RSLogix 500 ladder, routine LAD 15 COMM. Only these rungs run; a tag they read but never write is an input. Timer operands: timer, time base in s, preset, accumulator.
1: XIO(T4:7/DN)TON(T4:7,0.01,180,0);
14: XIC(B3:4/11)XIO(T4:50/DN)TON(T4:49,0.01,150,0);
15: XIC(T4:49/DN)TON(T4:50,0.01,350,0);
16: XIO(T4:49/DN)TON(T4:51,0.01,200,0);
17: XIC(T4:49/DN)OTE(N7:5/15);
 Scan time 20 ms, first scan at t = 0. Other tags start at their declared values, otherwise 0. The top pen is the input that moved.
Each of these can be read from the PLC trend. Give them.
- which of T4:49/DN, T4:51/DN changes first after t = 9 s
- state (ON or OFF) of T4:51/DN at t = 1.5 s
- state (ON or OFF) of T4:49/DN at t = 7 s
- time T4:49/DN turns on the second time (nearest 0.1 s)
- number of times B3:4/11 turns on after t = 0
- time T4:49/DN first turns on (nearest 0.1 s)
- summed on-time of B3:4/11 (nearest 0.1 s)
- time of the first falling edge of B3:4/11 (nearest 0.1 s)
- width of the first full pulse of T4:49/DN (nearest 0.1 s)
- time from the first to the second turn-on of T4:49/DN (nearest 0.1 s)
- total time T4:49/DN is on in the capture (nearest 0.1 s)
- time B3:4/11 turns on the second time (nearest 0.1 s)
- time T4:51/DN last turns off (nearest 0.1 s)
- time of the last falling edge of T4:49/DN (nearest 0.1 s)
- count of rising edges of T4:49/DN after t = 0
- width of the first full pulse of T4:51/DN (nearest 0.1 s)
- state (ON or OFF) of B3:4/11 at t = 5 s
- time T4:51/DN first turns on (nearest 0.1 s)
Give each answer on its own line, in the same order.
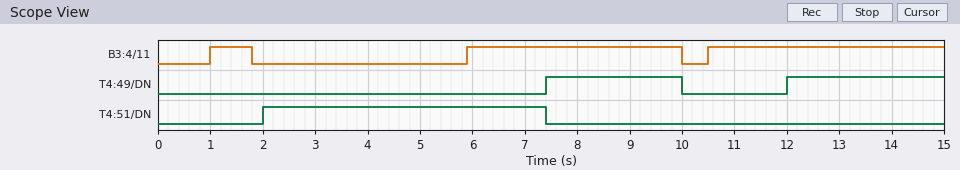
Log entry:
T4:49/DN
OFF
OFF
12.0 s
3
7.4 s
9.4 s
1.8 s
2.6 s
4.6 s
5.6 s
5.9 s
7.4 s
10.0 s
2
5.4 s
OFF
2.0 s
